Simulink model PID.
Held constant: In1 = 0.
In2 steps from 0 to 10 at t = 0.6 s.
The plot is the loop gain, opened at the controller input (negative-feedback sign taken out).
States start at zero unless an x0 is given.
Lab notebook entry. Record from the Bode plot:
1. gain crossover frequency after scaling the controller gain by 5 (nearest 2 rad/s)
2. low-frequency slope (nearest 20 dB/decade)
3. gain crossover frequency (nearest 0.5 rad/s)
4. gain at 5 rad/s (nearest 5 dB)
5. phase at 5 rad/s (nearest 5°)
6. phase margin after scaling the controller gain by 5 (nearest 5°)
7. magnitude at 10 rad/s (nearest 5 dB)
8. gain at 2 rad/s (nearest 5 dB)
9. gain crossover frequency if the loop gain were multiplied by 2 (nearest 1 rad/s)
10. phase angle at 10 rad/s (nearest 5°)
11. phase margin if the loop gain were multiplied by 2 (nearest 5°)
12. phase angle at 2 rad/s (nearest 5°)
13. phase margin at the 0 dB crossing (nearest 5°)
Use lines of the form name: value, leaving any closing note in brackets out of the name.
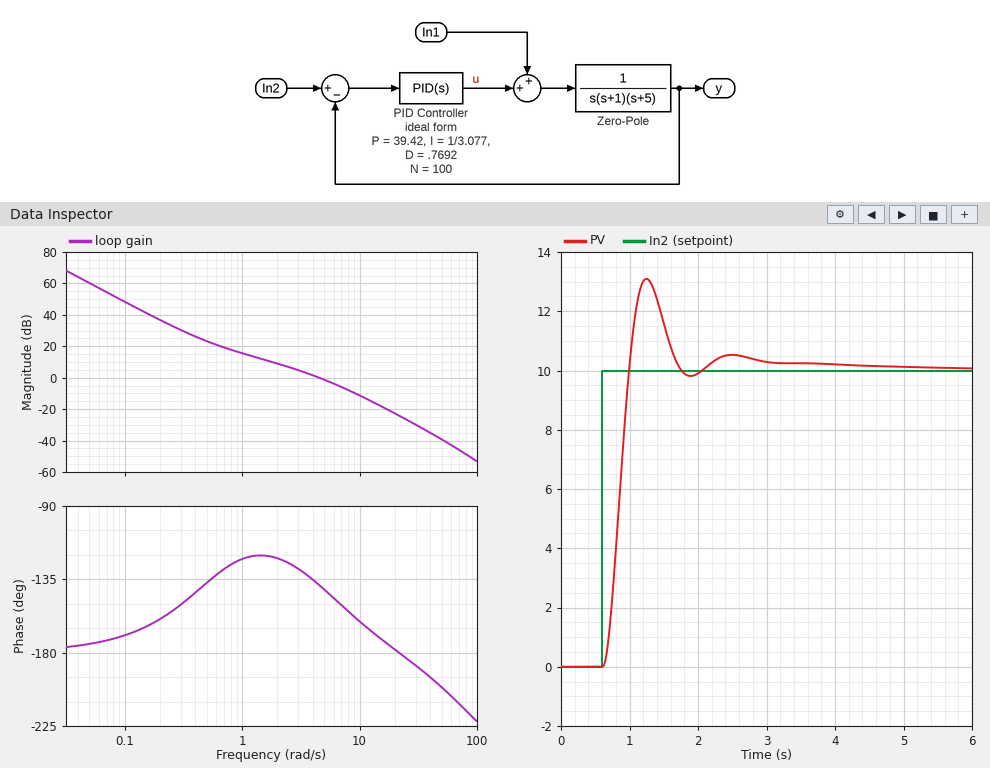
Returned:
gain crossover frequency after scaling the controller gain by 5: 12 rad/s
low-frequency slope: -40 dB/decade
gain crossover frequency: 4.5 rad/s
gain at 5 rad/s: 0 dB
phase at 5 rad/s: -140°
phase margin after scaling the controller gain by 5: 15°
magnitude at 10 rad/s: -10 dB
gain at 2 rad/s: 10 dB
gain crossover frequency if the loop gain were multiplied by 2: 7 rad/s
phase angle at 10 rad/s: -160°
phase margin if the loop gain were multiplied by 2: 30°
phase angle at 2 rad/s: -120°
phase margin at the 0 dB crossing: 40°
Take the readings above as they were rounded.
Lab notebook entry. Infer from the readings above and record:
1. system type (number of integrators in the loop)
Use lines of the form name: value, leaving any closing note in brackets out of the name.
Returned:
system type: 2
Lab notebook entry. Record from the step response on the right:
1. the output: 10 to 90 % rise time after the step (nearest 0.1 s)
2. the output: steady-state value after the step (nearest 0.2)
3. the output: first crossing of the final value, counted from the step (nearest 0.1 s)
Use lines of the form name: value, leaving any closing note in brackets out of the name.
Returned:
the output: 10 to 90 % rise time after the step: 0.3 s
the output: steady-state value after the step: 10.0
the output: first crossing of the final value, counted from the step: 0.4 s
